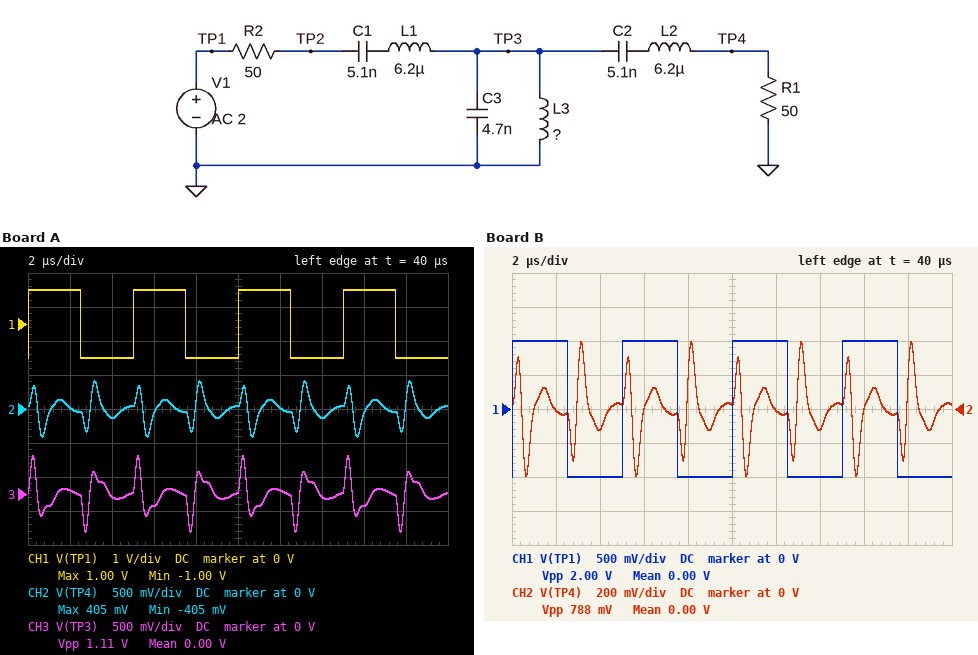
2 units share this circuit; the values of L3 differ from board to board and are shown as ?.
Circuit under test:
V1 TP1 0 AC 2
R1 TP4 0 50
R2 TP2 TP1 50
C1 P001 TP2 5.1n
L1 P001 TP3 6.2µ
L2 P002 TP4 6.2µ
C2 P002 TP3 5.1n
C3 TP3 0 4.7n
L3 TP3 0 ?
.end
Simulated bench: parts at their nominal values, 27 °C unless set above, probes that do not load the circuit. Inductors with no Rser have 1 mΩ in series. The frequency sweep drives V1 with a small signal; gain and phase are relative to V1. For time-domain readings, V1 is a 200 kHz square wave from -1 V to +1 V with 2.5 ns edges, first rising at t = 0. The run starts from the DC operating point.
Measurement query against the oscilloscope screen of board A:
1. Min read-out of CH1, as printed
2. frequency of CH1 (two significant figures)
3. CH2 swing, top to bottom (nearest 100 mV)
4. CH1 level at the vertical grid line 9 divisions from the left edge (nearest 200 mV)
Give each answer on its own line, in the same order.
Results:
-1.00 V
200 kHz
800 mV
-1.0 V
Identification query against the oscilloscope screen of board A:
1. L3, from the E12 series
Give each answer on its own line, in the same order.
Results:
4.7 µH
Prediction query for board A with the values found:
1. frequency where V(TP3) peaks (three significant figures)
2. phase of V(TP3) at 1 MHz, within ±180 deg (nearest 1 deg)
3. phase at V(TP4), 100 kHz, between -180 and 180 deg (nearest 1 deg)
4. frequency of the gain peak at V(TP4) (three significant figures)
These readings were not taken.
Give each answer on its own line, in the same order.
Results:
1.60 MHz
6 deg
-109 deg
1.43 MHz
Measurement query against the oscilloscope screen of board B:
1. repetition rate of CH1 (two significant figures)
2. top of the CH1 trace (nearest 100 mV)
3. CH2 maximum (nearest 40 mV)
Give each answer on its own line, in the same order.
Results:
200 kHz
1.0 V
400 mV
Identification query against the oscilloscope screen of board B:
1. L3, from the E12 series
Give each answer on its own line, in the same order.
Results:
3.9 µH
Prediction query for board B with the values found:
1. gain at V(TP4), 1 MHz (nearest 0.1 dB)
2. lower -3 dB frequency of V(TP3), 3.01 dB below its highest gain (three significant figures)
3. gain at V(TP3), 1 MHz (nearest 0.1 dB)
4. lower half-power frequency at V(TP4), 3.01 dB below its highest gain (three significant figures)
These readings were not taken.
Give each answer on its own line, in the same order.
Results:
-6.8 dB
1.05 MHz
-6.7 dB
618 kHz
